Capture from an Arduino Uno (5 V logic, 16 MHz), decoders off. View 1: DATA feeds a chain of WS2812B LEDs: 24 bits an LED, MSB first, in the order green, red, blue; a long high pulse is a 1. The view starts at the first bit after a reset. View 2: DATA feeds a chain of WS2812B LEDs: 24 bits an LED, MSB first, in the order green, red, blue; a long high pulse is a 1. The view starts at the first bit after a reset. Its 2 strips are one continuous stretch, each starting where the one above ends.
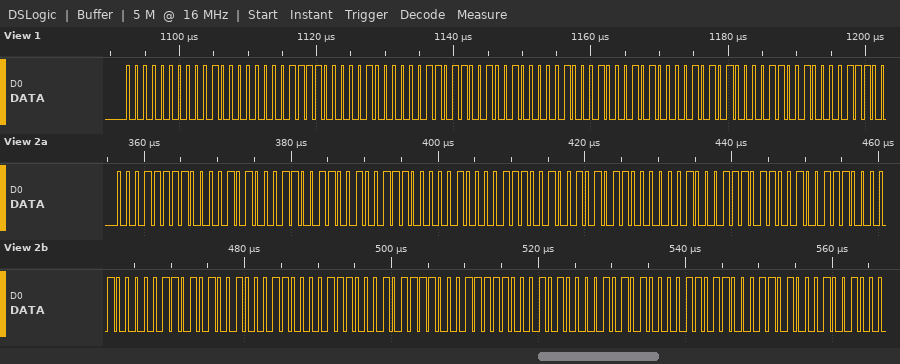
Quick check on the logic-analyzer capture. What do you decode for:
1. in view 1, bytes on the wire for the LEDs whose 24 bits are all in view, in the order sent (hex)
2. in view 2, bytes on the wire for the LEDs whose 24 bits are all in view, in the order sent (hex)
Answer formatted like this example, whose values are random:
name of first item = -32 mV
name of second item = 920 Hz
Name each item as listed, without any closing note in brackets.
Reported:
in view 1, bytes on the wire for the LEDs whose 24 bits are all in view, in the order sent = 00 20 1E 08 1B 24 11 14 2A
in view 2, bytes on the wire for the LEDs whose 24 bits are all in view, in the order sent = 1F 0A 33 27 04 39 2B 02 3B 27 08 35 23 0E 2F 1F 14 2A 1B 1A 24
